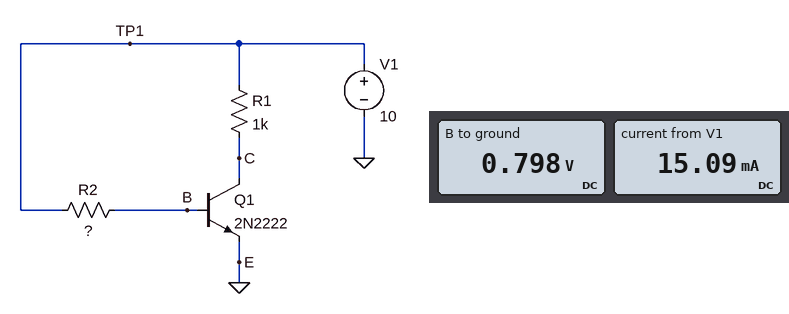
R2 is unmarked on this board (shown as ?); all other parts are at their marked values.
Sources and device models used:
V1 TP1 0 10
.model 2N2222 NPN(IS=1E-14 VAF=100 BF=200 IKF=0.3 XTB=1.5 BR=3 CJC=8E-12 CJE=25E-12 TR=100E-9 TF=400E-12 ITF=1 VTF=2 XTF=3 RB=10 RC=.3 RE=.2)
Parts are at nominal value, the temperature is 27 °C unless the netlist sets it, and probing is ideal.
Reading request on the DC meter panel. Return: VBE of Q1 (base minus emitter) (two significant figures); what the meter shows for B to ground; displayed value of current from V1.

800 mV
0.798 V
15.09 mA
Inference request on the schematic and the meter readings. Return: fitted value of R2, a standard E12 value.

1.8 kΩ
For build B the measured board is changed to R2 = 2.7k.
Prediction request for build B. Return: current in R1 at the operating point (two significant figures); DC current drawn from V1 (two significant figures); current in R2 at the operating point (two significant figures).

10 mA
13 mA
3.4 mA
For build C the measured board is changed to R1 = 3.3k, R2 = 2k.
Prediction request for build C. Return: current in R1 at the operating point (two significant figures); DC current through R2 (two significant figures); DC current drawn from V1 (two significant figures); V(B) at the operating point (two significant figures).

3.0 mA
4.6 mA
7.6 mA
780 mV
